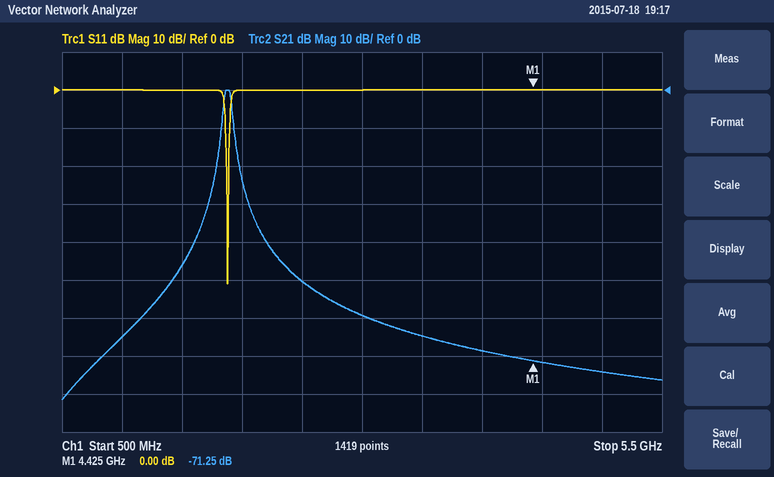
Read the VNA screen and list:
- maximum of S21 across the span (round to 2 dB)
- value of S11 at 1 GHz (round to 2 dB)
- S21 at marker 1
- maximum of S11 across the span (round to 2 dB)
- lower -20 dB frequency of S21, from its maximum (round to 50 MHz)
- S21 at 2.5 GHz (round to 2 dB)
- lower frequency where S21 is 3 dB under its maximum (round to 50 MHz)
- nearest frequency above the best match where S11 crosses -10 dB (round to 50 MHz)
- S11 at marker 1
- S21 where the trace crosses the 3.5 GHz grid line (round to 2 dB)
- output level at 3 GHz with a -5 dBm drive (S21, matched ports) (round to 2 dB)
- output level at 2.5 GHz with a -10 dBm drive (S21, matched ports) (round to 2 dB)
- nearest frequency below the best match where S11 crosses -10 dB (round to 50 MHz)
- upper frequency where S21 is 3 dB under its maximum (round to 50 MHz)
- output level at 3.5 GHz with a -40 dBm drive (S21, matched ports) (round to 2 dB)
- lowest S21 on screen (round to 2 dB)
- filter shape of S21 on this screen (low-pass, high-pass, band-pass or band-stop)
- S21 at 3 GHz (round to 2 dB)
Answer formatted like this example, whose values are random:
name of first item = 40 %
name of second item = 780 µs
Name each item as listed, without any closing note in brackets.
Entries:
maximum of S21 across the span = 0 dB
value of S11 at 1 GHz = 0 dB
S21 at marker 1 = -71.25 dB
maximum of S11 across the span = 0 dB
lower -20 dB frequency of S21, from its maximum = 1.80 GHz
S21 at 2.5 GHz = -50 dB
lower frequency where S21 is 3 dB under its maximum = 1.85 GHz
nearest frequency above the best match where S11 crosses -10 dB = 1.90 GHz
S11 at marker 1 = 0.00 dB
S21 where the trace crosses the 3.5 GHz grid line = -64 dB
output level at 3 GHz with a -5 dBm drive (S21, matched ports) = -64 dBm
output level at 2.5 GHz with a -10 dBm drive (S21, matched ports) = -60 dBm
nearest frequency below the best match where S11 crosses -10 dB = 1.85 GHz
upper frequency where S21 is 3 dB under its maximum = 1.90 GHz
output level at 3.5 GHz with a -40 dBm drive (S21, matched ports) = -104 dBm
lowest S21 on screen = -82 dB
filter shape of S21 on this screen = band-pass
S21 at 3 GHz = -60 dB
